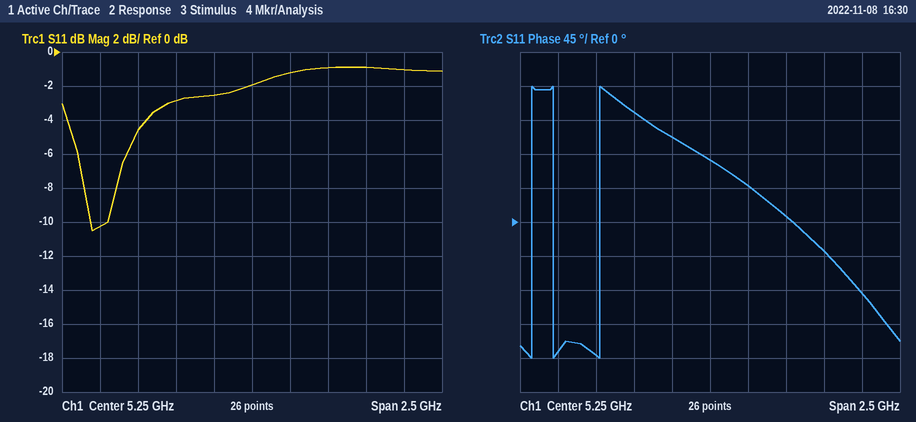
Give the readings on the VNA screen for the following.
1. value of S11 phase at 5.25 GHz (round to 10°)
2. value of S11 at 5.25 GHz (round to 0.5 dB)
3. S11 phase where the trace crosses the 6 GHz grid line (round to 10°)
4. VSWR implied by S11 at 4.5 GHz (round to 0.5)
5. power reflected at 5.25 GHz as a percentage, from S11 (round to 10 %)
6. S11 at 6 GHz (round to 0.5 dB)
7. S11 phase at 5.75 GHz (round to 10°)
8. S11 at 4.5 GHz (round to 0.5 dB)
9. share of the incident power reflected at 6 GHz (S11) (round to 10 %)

80°
-2.0 dB
-40°
4.0
60 %
-1.0 dB
10°
-4.5 dB
80 %
